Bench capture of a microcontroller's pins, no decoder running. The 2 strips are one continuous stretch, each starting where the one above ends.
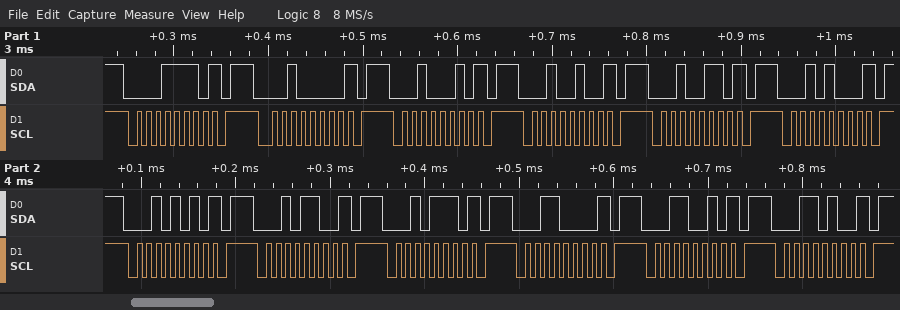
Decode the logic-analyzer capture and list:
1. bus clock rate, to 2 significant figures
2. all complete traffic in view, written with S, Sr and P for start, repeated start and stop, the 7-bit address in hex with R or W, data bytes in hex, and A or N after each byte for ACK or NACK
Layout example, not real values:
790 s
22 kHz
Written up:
100 kHz
S 0FW N P S 10W N P S 11W N P S 12W N P S 13W N P S 14W N P S 15W N P S 16W N P S 17W N P S 18W N P S 19W N P S 1AW N P
